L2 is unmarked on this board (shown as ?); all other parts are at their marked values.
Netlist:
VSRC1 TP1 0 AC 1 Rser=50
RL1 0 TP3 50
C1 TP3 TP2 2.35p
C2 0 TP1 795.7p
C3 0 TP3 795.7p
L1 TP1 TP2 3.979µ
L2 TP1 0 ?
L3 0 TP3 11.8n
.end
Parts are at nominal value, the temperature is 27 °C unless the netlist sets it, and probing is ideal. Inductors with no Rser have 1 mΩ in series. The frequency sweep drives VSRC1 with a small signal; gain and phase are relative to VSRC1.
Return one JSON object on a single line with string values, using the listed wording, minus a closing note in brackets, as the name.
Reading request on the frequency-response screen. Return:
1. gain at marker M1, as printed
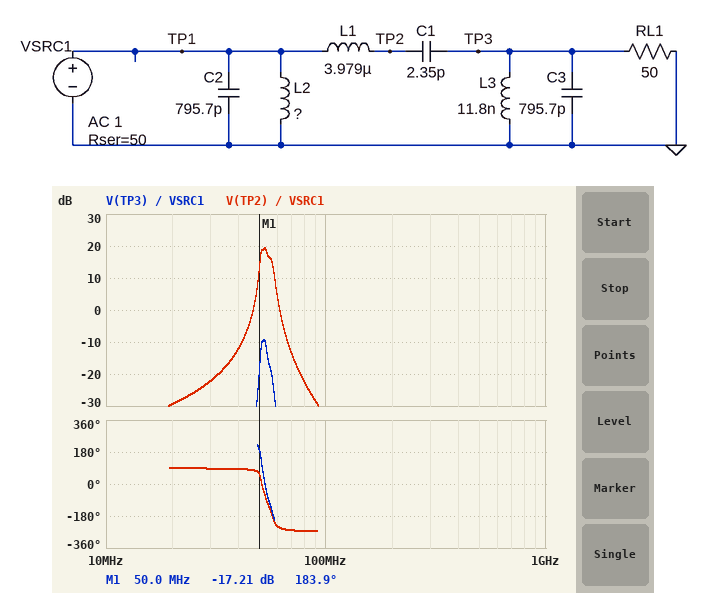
{"gain at marker M1, as printed": "-17.21 dB"}
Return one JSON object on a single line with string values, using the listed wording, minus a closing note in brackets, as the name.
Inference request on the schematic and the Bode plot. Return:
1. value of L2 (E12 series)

{"value of L2": "10 nH"}
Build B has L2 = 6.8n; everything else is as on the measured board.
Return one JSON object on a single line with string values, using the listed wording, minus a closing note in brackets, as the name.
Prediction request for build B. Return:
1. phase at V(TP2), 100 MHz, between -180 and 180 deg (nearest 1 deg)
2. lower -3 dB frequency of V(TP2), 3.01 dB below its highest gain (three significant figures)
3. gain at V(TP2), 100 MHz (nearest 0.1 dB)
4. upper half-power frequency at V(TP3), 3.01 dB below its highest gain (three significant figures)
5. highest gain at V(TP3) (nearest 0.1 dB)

{"phase at V(TP2), 100 MHz, between -180 and 180 deg": "94 deg", "lower -3 dB frequency of V(TP2), 3.01 dB below its highest gain": "50.5 MHz", "gain at V(TP2), 100 MHz": "-31.0 dB", "upper half-power frequency at V(TP3), 3.01 dB below its highest gain": "53.5 MHz", "highest gain at V(TP3)": "-19.5 dB"}
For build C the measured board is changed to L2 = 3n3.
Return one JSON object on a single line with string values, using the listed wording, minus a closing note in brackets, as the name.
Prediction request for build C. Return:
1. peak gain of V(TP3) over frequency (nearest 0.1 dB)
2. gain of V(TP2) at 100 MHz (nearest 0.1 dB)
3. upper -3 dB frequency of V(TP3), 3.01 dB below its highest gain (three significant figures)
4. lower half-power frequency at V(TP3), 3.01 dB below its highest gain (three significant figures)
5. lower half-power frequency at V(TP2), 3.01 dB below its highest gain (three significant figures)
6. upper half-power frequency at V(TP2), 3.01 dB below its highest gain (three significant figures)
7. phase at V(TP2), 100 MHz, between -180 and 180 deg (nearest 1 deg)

{"peak gain of V(TP3) over frequency": "-30.3 dB", "gain of V(TP2) at 100 MHz": "-11.0 dB", "upper -3 dB frequency of V(TP3), 3.01 dB below its highest gain": "53.5 MHz", "lower half-power frequency at V(TP3), 3.01 dB below its highest gain": "50.7 MHz", "lower half-power frequency at V(TP2), 3.01 dB below its highest gain": "50.5 MHz", "upper half-power frequency at V(TP2), 3.01 dB below its highest gain": "53.8 MHz", "phase at V(TP2), 100 MHz, between -180 and 180 deg": "140 deg"}
